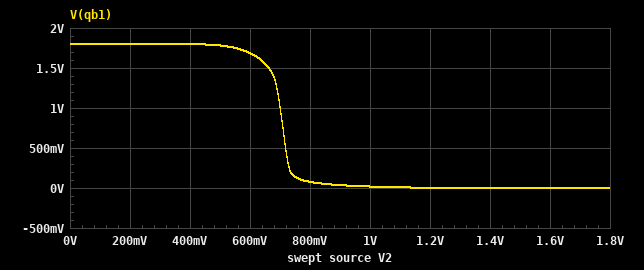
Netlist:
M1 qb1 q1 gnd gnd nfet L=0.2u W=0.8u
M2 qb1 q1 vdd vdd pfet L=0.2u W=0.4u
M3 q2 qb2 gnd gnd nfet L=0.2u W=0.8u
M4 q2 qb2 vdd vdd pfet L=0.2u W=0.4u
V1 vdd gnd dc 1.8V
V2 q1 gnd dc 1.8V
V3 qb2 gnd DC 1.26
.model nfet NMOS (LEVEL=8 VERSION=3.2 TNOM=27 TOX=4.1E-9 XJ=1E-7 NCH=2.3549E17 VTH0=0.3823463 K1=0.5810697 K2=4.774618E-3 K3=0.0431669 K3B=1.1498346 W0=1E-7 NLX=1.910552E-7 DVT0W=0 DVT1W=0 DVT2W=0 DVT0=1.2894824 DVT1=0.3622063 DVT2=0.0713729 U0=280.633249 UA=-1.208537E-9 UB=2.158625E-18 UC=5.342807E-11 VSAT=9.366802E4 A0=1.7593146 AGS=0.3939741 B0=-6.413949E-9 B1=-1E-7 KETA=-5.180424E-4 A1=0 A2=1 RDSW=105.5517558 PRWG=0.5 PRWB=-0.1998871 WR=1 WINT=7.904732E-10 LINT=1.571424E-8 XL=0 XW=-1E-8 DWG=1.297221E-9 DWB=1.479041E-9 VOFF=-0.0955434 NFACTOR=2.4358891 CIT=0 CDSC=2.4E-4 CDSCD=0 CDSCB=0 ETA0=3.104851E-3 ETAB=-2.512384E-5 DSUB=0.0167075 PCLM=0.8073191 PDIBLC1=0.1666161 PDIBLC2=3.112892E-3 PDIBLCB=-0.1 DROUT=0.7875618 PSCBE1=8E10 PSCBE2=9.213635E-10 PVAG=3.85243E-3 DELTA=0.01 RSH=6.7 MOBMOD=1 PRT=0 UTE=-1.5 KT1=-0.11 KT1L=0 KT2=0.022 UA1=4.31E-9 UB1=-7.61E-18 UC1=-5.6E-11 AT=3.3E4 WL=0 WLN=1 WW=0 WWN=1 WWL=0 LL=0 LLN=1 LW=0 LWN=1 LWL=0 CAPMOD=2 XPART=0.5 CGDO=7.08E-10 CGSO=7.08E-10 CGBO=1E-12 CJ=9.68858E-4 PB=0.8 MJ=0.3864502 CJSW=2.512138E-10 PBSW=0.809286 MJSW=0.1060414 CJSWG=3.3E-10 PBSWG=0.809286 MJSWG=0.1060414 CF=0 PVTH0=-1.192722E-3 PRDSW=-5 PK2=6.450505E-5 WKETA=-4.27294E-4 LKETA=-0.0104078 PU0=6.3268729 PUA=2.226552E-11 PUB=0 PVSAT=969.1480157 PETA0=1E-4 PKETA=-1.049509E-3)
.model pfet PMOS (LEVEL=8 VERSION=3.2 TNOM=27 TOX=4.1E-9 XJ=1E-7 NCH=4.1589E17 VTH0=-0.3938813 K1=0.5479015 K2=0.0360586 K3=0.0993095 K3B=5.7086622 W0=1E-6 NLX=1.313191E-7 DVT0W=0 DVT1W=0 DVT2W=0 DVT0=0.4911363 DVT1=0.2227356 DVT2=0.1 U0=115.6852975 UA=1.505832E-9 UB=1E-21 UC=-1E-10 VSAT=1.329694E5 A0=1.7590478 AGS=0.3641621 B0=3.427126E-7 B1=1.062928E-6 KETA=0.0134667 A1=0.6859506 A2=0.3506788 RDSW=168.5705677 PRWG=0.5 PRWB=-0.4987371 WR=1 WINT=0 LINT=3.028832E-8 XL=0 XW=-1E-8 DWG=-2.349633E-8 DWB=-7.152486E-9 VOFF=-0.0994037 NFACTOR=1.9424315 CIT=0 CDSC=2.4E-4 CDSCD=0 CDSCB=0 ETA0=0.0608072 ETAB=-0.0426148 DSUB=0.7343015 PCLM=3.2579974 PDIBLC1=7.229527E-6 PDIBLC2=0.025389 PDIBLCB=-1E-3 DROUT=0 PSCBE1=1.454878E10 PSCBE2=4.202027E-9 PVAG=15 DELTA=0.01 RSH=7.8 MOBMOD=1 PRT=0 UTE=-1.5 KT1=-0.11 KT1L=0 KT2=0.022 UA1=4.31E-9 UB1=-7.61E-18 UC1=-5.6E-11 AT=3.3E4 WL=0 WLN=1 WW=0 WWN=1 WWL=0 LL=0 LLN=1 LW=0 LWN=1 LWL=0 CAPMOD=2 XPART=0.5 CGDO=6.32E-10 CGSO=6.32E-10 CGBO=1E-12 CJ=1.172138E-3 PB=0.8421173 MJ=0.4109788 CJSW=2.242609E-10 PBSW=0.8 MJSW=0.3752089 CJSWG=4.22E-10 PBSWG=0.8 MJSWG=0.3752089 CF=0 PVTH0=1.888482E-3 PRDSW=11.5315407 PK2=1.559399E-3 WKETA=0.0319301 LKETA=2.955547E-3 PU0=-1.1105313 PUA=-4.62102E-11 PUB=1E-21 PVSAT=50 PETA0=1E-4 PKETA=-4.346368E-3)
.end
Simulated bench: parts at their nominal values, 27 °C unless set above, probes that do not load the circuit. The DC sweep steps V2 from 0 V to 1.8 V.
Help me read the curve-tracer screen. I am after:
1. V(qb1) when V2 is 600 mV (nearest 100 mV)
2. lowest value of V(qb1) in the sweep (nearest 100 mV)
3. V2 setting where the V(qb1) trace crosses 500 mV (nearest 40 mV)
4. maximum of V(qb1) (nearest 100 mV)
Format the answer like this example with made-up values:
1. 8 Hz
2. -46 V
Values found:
1. 1.7 V
2. 0 V
3. 720 mV
4. 1.8 V
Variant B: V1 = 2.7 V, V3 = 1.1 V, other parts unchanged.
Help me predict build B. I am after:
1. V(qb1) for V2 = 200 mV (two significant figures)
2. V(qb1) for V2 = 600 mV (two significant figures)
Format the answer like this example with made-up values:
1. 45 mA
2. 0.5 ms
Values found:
1. 2.7 V
2. 2.6 V
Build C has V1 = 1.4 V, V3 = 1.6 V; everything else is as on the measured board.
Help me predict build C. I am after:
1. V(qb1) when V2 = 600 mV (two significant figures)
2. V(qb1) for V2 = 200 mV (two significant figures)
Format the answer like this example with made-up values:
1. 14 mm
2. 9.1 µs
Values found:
1. 840 mV
2. 1.4 V
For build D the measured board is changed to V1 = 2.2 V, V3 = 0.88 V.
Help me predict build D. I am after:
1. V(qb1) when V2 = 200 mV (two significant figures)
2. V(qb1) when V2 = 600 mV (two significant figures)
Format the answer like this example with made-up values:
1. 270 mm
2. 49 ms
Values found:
1. 2.2 V
2. 2.1 V
